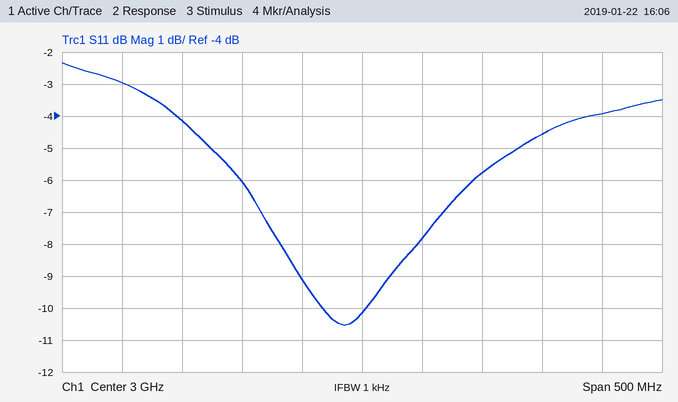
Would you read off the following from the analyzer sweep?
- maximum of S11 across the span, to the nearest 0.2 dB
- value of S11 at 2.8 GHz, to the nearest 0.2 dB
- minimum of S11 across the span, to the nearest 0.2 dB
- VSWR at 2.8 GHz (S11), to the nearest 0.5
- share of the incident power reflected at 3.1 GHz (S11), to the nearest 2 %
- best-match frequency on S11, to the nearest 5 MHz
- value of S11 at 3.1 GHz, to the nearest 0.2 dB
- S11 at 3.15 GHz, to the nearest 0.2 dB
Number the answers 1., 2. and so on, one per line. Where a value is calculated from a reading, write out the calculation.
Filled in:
1. -2.4 dB
2. -3.0 dB
3. -10.6 dB
4. |Γ| = 10^(-3/20) = 0.7079; VSWR = (1 + 0.7079)/(1 − 0.7079) ≈ 5.85, so 6.0 to the nearest 0.5
5. 10^(-5.8/10) ≈ 26 %
6. 2.985 GHz
7. -5.8 dB
8. -4.6 dB
